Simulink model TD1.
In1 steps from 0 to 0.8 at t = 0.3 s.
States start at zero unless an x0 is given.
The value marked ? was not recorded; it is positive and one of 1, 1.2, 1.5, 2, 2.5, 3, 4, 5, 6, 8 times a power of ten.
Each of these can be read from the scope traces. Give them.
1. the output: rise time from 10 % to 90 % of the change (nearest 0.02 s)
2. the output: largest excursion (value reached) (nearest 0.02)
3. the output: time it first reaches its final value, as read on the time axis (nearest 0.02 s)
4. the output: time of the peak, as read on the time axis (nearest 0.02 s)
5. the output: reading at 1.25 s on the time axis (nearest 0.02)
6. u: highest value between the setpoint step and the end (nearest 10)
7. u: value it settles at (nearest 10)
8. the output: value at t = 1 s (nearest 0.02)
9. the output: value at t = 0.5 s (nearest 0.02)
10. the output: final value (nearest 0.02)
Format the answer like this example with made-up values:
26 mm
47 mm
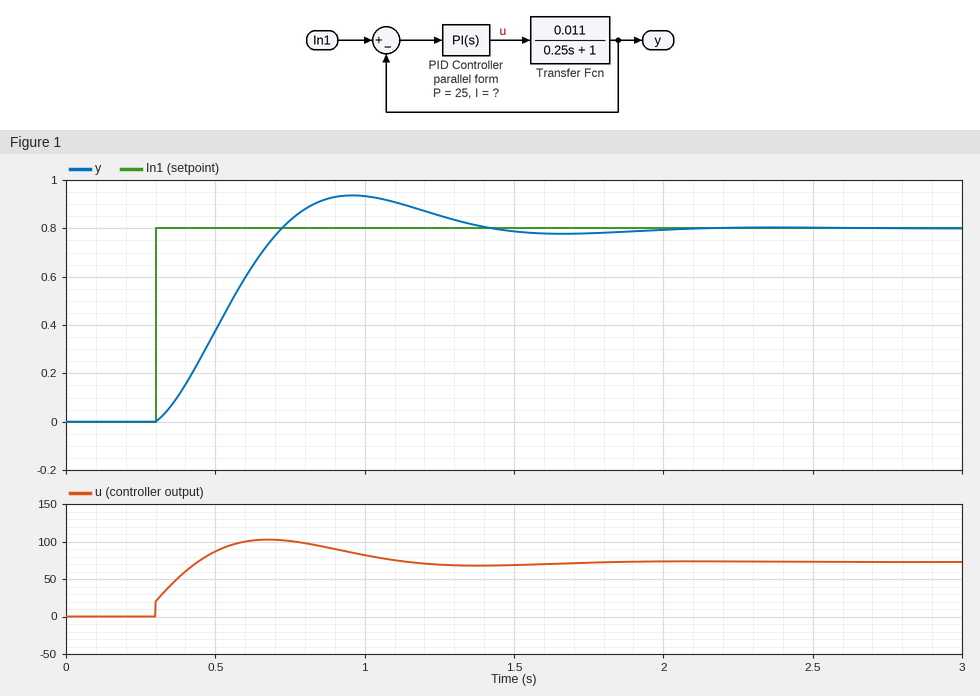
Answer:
0.30 s
0.94
0.72 s
0.96 s
0.86
100
70
0.94
0.38
0.80
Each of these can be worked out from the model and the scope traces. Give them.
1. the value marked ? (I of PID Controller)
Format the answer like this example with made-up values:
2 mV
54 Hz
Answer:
600
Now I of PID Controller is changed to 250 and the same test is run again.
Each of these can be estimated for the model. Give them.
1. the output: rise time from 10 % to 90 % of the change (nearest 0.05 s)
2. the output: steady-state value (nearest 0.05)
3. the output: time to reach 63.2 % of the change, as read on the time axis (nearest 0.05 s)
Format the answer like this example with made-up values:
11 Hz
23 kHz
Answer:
0.65 s
0.80
0.75 s
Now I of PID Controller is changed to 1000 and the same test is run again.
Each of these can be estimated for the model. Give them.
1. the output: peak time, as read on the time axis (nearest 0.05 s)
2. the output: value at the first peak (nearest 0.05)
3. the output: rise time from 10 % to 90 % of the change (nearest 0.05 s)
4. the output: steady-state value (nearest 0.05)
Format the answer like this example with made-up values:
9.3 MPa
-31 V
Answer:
0.80 s
1.00
0.20 s
0.80
